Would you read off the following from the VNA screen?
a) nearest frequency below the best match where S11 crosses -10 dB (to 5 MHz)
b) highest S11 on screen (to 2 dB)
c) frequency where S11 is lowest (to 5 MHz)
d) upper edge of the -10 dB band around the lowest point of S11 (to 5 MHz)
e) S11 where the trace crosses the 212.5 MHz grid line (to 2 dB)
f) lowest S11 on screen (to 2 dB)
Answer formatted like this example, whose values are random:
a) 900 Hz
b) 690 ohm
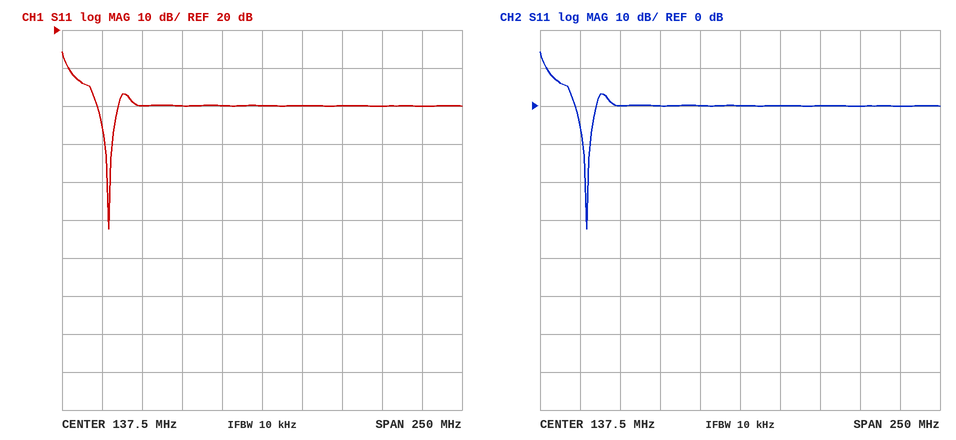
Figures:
a) 40 MHz
b) 14 dB
c) 40 MHz
d) 45 MHz
e) 0 dB
f) -32 dB
